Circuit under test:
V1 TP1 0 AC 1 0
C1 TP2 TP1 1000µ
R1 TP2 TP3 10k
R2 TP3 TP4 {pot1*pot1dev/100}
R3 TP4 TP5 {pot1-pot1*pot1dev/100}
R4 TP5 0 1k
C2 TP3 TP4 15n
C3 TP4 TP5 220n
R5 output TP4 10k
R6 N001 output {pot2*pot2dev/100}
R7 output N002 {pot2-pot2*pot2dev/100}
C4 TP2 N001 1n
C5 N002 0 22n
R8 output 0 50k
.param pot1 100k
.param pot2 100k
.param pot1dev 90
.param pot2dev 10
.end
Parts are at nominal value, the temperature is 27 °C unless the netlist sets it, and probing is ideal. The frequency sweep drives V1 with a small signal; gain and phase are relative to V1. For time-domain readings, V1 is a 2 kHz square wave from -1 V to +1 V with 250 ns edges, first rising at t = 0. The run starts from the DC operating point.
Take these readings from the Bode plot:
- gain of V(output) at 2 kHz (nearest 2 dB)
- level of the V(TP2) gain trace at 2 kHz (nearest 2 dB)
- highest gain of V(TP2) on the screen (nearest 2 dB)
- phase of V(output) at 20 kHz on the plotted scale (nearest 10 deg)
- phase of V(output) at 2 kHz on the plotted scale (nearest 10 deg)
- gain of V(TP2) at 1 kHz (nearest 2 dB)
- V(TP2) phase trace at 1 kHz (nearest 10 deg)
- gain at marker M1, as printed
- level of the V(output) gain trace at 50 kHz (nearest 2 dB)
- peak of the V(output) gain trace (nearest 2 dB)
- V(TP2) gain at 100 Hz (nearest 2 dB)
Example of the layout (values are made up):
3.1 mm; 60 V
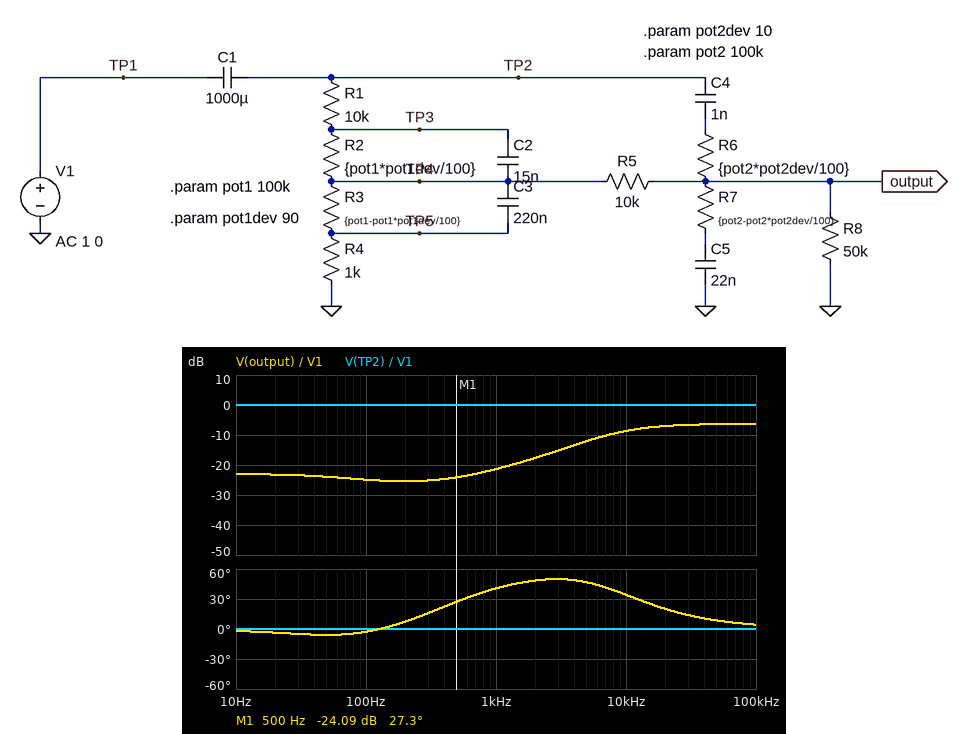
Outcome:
-18 dB; 0 dB; 0 dB; 20 deg; 50 deg; 0 dB; 0 deg; -24.09 dB; -6 dB; -6 dB; 0 dB
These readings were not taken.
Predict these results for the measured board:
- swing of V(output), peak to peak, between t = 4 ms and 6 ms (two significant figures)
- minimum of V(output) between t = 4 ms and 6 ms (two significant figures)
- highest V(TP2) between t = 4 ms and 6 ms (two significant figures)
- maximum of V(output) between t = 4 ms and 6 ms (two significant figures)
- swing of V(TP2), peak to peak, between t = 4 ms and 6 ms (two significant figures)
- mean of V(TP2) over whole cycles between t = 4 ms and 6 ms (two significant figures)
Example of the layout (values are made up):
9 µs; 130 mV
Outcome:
1.8 V; -840 mV; 2.0 V; 980 mV; 2.0 V; 1.0 V
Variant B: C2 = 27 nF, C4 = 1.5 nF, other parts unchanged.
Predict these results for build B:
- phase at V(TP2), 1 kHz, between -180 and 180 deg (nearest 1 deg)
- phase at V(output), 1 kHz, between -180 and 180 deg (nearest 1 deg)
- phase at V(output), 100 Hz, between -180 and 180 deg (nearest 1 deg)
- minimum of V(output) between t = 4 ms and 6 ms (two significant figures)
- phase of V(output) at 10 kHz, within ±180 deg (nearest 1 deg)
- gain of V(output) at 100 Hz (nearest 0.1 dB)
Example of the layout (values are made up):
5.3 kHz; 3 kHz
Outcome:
0 deg; 36 deg; 9 deg; -820 mV; 25 deg; -22.1 dB
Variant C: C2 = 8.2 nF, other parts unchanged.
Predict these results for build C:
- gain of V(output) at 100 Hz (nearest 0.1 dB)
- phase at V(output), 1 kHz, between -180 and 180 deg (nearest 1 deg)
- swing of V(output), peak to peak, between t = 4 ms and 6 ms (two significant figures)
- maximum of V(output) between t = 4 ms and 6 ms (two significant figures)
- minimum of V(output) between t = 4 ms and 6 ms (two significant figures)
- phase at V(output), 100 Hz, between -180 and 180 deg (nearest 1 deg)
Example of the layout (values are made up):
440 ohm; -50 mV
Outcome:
-26.5 dB; 53 deg; 1.9 V; 1.0 V; -860 mV; -14 deg
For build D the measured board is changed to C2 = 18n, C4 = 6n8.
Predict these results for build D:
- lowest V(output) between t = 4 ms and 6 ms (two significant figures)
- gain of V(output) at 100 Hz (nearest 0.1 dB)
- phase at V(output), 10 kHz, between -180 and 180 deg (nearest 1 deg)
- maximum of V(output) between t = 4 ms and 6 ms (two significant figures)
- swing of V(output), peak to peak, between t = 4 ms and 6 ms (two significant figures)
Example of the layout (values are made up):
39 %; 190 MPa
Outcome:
-730 mV; -21.8 dB; 6 deg; 870 mV; 1.6 V
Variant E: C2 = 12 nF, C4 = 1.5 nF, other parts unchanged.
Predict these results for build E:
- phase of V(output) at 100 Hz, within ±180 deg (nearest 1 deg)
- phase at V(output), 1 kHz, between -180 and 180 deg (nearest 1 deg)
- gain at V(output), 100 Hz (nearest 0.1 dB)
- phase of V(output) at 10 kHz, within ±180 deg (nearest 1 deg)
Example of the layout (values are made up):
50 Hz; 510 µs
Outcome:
-4 deg; 51 deg; -25.5 dB; 26 deg
